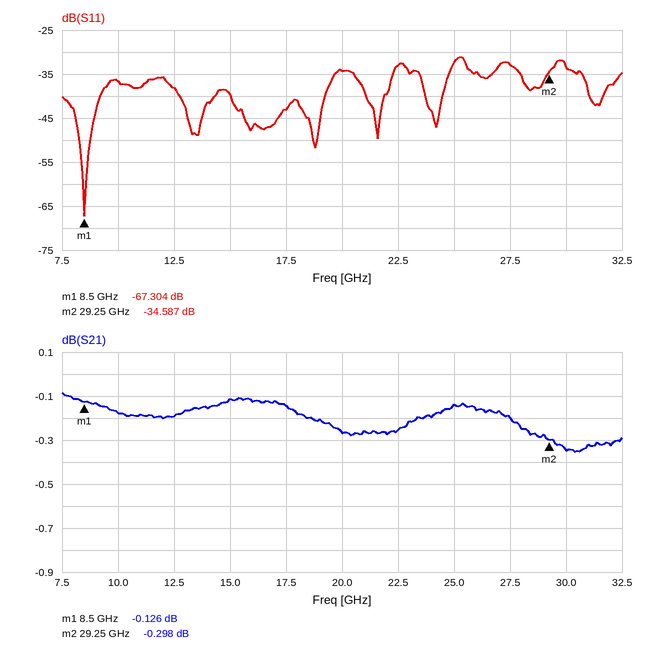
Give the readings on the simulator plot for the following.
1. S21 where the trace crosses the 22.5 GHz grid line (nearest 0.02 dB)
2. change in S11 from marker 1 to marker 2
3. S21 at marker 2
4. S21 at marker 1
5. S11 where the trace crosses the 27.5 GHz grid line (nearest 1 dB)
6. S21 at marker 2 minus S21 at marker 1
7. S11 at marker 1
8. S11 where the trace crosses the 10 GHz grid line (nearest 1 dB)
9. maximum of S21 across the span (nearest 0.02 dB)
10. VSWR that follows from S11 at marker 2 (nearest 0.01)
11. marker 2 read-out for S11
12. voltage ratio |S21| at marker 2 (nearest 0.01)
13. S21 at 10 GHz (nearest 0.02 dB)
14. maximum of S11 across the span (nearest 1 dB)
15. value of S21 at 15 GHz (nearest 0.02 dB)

-0.26 dB
32.717 dB
-0.298 dB
-0.126 dB
-33 dB
-0.172 dB
-67.304 dB
-37 dB
-0.08 dB
1.04
-34.587 dB
0.97
-0.18 dB
-31 dB
-0.12 dB
